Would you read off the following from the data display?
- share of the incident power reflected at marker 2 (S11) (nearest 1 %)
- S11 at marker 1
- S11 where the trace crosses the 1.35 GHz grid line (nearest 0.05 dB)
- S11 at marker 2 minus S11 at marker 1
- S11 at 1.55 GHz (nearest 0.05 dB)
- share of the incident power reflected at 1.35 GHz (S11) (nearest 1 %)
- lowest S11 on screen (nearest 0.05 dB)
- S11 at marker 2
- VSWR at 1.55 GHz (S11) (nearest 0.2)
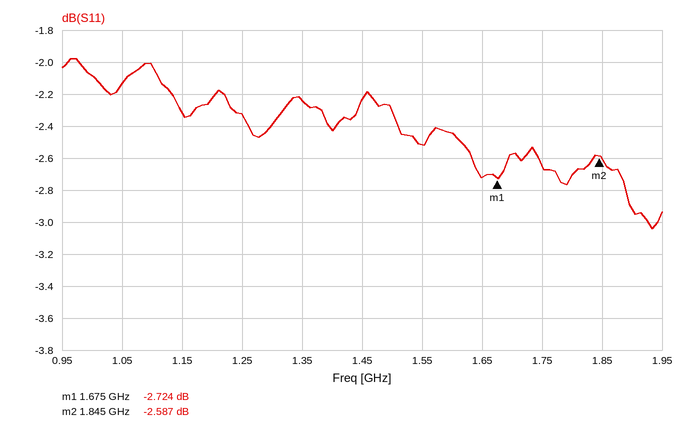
55 %
-2.724 dB
-2.25 dB
0.137 dB
-2.50 dB
60 %
-3.05 dB
-2.587 dB
7.0
